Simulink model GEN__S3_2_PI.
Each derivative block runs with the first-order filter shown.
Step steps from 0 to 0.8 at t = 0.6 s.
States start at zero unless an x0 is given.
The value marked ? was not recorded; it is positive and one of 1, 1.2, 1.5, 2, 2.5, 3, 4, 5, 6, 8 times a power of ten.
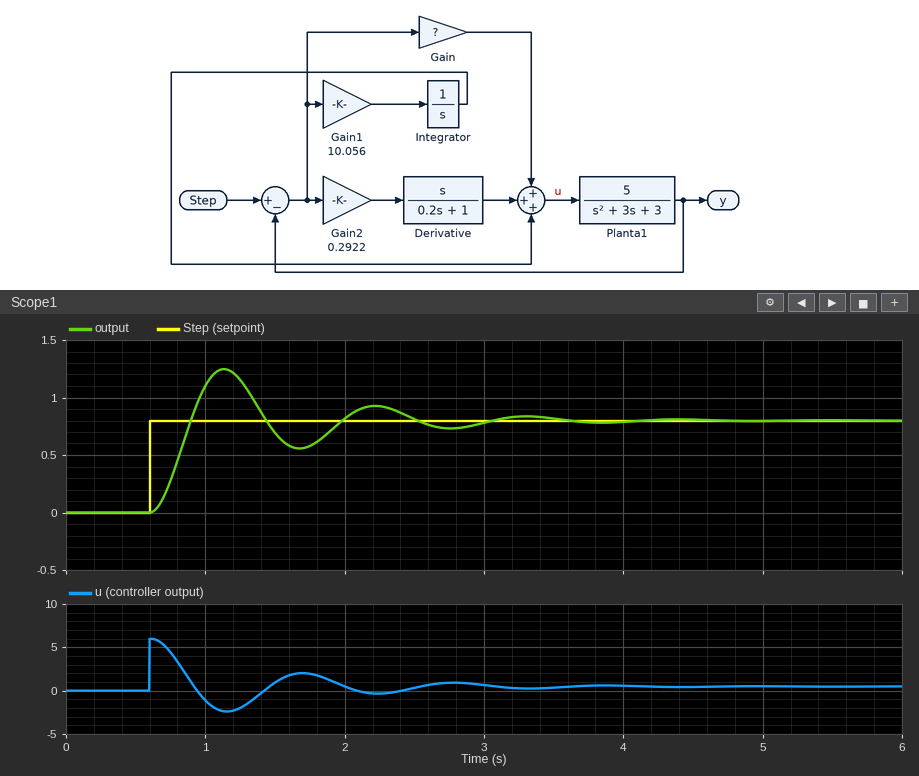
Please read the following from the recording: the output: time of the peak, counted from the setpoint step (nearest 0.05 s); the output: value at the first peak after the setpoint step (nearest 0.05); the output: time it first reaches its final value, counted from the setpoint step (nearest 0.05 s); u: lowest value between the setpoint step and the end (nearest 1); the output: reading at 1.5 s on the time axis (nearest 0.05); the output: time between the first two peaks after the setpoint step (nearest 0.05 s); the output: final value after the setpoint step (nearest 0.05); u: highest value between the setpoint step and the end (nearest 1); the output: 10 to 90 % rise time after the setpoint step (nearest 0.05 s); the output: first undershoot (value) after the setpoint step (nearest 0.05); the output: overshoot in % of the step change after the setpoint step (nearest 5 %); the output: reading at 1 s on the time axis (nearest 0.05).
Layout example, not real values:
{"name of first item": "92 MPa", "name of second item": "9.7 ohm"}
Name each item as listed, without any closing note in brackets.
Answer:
{"the output: time of the peak, counted from the setpoint step": "0.55 s", "the output: value at the first peak after the setpoint step": "1.25", "the output: time it first reaches its final value, counted from the setpoint step": "0.30 s", "u: lowest value between the setpoint step and the end": "-2", "the output: reading at 1.5 s on the time axis": "0.70", "the output: time between the first two peaks after the setpoint step": "1.10 s", "the output: final value after the setpoint step": "0.80", "u: highest value between the setpoint step and the end": "6", "the output: 10 to 90 % rise time after the setpoint step": "0.20 s", "the output: first undershoot (value) after the setpoint step": "0.55", "the output: overshoot in % of the step change after the setpoint step": "55 %", "the output: reading at 1 s on the time axis": "1.10"}
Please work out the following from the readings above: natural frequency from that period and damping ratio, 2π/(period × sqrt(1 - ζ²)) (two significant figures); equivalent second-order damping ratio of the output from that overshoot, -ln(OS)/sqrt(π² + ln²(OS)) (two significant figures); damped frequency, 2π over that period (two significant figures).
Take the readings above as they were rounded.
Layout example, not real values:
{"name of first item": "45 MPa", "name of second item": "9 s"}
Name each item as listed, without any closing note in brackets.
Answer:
{"natural frequency from that period and damping ratio, 2π/(period × sqrt(1 - ζ²))": "5.8 rad/s", "equivalent second-order damping ratio of the output from that overshoot, -ln(OS)/sqrt(π² + ln²(OS))": "0.19", "damped frequency, 2π over that period": "5.7 rad/s"}
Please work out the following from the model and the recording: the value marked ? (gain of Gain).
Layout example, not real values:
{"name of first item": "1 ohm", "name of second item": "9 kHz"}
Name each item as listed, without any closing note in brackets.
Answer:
{"the value marked ?": "6"}
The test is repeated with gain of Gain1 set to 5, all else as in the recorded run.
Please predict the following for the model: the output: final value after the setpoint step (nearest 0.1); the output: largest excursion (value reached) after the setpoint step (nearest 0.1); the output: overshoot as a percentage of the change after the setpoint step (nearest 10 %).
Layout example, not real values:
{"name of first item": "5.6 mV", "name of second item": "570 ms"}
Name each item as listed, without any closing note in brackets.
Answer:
{"the output: final value after the setpoint step": "0.8", "the output: largest excursion (value reached) after the setpoint step": "1.1", "the output: overshoot as a percentage of the change after the setpoint step": "40 %"}
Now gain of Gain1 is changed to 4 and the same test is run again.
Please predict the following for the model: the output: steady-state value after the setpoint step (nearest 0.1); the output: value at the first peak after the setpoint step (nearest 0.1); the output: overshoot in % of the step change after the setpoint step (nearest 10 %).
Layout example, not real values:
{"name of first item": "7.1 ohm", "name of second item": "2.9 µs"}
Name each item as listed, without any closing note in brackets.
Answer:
{"the output: steady-state value after the setpoint step": "0.8", "the output: value at the first peak after the setpoint step": "1.1", "the output: overshoot in % of the step change after the setpoint step": "40 %"}
